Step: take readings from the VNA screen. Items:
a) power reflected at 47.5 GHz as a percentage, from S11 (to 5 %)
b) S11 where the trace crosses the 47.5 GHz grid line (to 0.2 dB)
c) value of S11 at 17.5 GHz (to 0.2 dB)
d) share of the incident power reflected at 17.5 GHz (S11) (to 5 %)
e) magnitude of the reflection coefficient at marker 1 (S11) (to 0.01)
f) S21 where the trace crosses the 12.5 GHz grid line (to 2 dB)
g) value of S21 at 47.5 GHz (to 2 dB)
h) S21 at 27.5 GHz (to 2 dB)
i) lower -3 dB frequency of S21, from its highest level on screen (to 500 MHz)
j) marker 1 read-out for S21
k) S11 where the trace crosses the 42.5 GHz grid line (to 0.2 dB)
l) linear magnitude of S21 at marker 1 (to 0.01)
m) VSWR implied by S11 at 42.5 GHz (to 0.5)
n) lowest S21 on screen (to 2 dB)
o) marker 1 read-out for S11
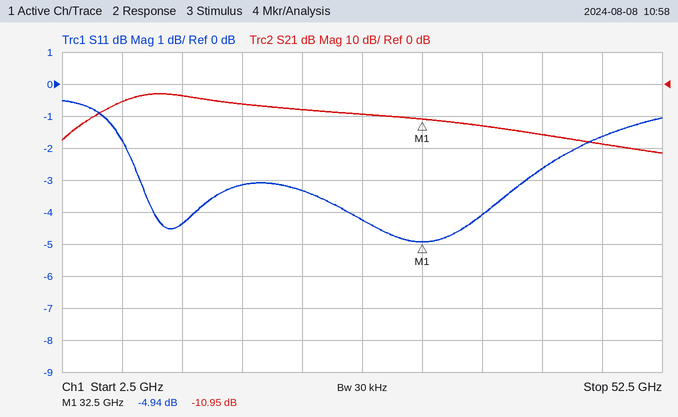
70 %
-1.6 dB
-3.2 dB
50 %
0.57
-4 dB
-18 dB
-10 dB
7.0 GHz
-10.95 dB
-2.6 dB
0.28
6.5
-22 dB
-4.94 dB
